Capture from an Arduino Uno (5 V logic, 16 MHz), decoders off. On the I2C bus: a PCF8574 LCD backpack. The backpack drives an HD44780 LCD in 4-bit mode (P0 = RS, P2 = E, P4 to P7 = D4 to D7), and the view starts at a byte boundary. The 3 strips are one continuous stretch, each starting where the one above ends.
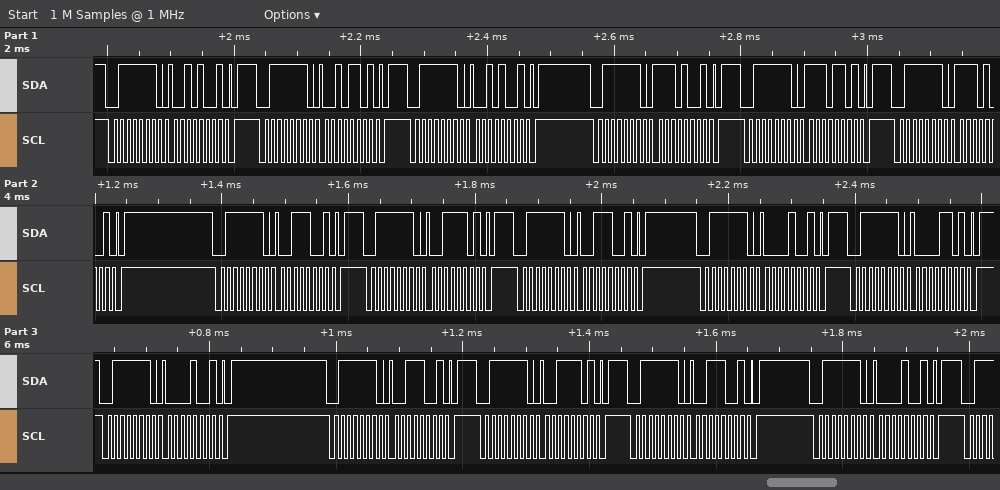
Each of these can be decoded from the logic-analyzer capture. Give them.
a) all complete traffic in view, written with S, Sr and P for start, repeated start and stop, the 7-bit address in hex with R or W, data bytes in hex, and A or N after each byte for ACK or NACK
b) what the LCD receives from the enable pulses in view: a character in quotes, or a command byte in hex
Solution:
S 3FW A 29 A P S 3FW A 2D A P S 3FW A 29 A P S 3FW A E9 A P S 3FW A ED A P S 3FW A E9 A P S 3FW A 39 A P S 3FW A 3D A P S 3FW A 39 A P S 3FW A 09 A P S 3FW A 0D A P S 3FW A 09 A P S 3FW A 39 A P S 3FW A 3D A P S 3FW A 39 A P S 3FW A 09 A P
'.' '0'
